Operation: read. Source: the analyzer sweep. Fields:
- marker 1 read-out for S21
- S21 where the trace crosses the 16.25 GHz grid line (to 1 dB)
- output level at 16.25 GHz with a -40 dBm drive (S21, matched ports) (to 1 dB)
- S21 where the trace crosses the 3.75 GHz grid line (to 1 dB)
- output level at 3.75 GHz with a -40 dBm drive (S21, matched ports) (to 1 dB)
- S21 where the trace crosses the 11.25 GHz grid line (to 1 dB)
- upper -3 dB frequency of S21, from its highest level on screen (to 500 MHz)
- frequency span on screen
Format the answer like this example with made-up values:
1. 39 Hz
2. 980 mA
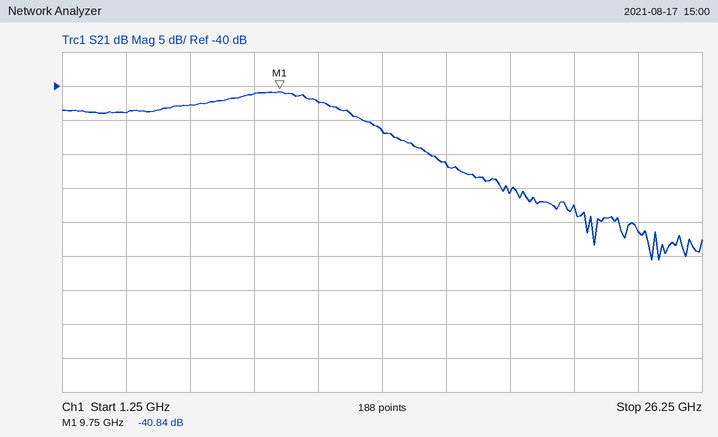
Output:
1. -40.84 dB
2. -51 dB
3. -91 dBm
4. -44 dB
5. -84 dBm
6. -42 dB
7. 12.5 GHz
8. 25 GHz
